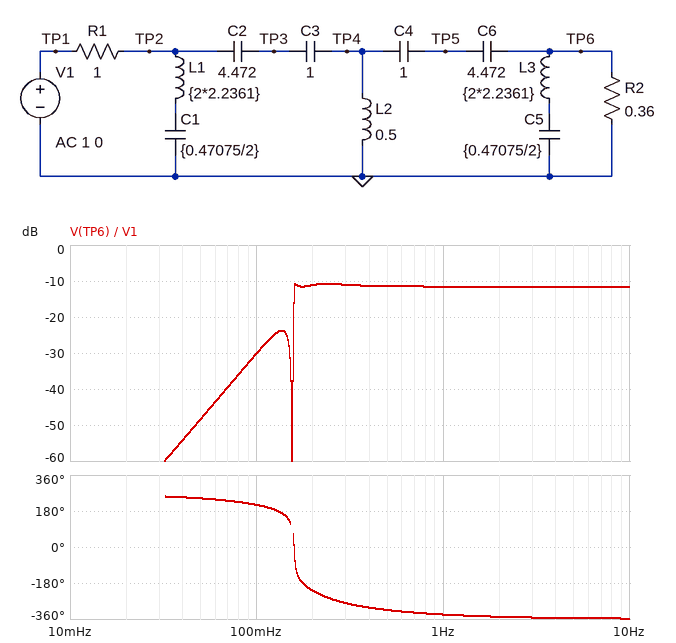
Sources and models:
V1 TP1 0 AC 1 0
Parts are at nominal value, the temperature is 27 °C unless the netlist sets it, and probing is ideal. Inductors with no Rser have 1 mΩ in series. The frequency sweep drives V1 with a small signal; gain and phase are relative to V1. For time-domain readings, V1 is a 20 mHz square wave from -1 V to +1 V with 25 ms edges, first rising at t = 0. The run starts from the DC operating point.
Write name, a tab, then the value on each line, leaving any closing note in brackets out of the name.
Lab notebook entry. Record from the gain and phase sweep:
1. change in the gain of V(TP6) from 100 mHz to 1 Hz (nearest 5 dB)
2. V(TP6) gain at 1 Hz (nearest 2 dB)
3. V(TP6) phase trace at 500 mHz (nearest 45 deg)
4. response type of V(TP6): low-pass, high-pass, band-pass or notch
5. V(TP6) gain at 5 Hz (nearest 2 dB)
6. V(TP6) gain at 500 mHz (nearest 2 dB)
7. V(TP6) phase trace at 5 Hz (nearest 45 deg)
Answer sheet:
change in the gain of V(TP6) from 100 mHz to 1 Hz	20 dB
V(TP6) gain at 1 Hz	-12 dB
V(TP6) phase trace at 500 mHz	-315 deg
response type of V(TP6): low-pass, high-pass, band-pass or notch	high-pass
V(TP6) gain at 5 Hz	-12 dB
V(TP6) gain at 500 mHz	-12 dB
V(TP6) phase trace at 5 Hz	-360 deg
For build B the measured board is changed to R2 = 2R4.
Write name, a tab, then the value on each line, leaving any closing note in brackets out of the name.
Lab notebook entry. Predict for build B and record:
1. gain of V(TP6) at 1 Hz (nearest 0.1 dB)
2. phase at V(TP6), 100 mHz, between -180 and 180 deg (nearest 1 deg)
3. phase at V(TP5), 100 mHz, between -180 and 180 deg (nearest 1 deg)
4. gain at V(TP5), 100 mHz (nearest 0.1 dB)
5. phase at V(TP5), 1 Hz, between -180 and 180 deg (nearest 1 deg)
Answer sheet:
gain of V(TP6) at 1 Hz	-3.0 dB
phase at V(TP6), 100 mHz, between -180 and 180 deg	164 deg
phase at V(TP5), 100 mHz, between -180 and 180 deg	156 deg
gain at V(TP5), 100 mHz	-19.8 dB
phase at V(TP5), 1 Hz, between -180 and 180 deg	22 deg
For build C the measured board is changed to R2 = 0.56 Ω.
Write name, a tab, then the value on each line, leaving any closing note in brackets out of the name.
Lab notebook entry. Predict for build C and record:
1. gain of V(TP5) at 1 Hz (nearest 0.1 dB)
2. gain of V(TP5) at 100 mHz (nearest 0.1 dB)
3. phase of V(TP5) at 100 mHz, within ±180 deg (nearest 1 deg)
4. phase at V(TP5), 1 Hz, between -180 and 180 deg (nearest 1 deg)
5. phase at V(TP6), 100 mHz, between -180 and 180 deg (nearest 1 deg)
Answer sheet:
gain of V(TP5) at 1 Hz	-8.9 dB
gain of V(TP5) at 100 mHz	-24.8 dB
phase of V(TP5) at 100 mHz, within ±180 deg	172 deg
phase at V(TP5), 1 Hz, between -180 and 180 deg	19 deg
phase at V(TP6), 100 mHz, between -180 and 180 deg	-158 deg
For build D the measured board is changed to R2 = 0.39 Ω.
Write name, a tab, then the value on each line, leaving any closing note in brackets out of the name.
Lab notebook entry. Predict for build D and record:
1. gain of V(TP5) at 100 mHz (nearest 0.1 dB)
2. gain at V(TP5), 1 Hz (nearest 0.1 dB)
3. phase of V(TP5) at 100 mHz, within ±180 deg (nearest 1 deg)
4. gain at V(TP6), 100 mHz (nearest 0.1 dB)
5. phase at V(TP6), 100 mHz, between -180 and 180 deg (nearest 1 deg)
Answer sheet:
gain of V(TP5) at 100 mHz	-26.4 dB
gain at V(TP5), 1 Hz	-11.0 dB
phase of V(TP5) at 100 mHz, within ±180 deg	169 deg
gain at V(TP6), 100 mHz	-29.5 dB
phase at V(TP6), 100 mHz, between -180 and 180 deg	-151 deg
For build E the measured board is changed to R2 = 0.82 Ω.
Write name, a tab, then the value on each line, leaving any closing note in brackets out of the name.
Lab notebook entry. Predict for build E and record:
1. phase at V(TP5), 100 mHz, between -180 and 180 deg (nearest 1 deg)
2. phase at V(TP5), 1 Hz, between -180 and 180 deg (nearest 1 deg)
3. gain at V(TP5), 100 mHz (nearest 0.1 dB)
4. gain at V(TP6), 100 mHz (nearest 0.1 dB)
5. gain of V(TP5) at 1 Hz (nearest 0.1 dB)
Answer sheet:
phase at V(TP5), 100 mHz, between -180 and 180 deg	171 deg
phase at V(TP5), 1 Hz, between -180 and 180 deg	20 deg
gain at V(TP5), 100 mHz	-23.0 dB
gain at V(TP6), 100 mHz	-24.4 dB
gain of V(TP5) at 1 Hz	-6.9 dB
